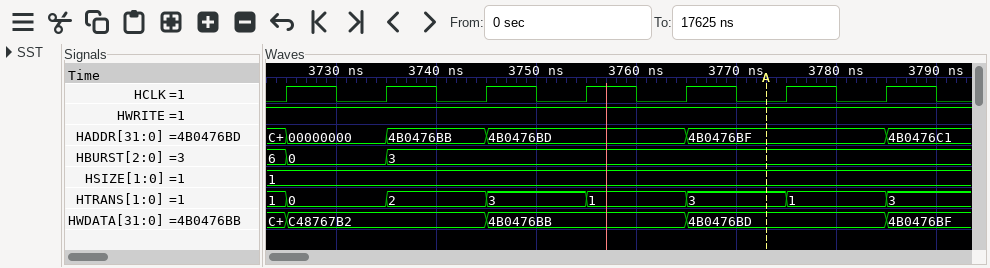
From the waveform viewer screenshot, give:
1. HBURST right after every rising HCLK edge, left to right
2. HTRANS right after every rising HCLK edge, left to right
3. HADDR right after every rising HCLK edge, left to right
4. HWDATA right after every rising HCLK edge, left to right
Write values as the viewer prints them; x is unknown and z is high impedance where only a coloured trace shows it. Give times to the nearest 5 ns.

0, 3, 3, 3, 3, 3, 3
0, 2, 3, 1, 3, 1, 3
00000000, 4B0476BB, 4B0476BD, 4B0476BD, 4B0476BF, 4B0476BF, 4B0476C1
C48767B2, C48767B2, 4B0476BB, 4B0476BB, 4B0476BD, 4B0476BD, 4B0476BF
